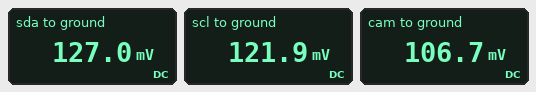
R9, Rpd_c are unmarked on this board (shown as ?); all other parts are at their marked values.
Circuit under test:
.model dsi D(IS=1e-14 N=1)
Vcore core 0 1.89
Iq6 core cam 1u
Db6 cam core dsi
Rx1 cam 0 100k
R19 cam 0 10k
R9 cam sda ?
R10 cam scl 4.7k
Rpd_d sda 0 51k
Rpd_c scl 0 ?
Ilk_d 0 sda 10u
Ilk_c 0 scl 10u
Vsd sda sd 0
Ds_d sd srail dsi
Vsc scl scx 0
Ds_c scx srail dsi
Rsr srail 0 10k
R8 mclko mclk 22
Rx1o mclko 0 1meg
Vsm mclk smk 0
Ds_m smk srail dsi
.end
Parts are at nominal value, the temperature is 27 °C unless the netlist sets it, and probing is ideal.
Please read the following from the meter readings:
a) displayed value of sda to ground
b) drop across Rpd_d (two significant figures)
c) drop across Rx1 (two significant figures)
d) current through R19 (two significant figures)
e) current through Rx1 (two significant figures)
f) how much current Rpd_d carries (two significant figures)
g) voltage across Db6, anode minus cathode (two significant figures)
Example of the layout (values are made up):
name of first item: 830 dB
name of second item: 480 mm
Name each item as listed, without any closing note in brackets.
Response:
displayed value of sda to ground: 127.0 mV
drop across Rpd_d: 130 mV
drop across Rx1: 110 mV
current through R19: 11 µA
current through Rx1: 1.1 µA
how much current Rpd_d carries: 2.5 µA
voltage across Db6, anode minus cathode: -1.8 V
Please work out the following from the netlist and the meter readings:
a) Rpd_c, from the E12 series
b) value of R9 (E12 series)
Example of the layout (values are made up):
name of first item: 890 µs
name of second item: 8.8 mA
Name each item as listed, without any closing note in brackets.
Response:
Rpd_c, from the E12 series: 18 kΩ
value of R9: 2.7 kΩ
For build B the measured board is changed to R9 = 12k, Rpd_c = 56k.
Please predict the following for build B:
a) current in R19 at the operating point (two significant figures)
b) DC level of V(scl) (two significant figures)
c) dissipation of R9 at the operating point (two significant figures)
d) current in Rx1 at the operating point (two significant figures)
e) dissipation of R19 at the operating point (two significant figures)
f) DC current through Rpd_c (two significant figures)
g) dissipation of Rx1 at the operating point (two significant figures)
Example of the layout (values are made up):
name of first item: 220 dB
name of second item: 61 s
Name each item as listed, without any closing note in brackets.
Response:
current in R19 at the operating point: 13 µA
DC level of V(scl): 160 mV
dissipation of R9 at the operating point: 440 nW
current in Rx1 at the operating point: 1.3 µA
dissipation of R19 at the operating point: 1.7 µW
DC current through Rpd_c: 2.9 µA
dissipation of Rx1 at the operating point: 170 nW
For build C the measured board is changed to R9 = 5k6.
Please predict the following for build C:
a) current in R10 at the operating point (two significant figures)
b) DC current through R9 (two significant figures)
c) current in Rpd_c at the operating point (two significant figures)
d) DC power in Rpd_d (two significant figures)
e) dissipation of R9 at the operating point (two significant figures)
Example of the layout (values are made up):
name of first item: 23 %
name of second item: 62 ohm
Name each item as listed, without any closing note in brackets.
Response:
current in R10 at the operating point: 3.3 µA
DC current through R9: 7.2 µA
current in Rpd_c at the operating point: 6.7 µA
DC power in Rpd_d: 410 nW
dissipation of R9 at the operating point: 290 nW
